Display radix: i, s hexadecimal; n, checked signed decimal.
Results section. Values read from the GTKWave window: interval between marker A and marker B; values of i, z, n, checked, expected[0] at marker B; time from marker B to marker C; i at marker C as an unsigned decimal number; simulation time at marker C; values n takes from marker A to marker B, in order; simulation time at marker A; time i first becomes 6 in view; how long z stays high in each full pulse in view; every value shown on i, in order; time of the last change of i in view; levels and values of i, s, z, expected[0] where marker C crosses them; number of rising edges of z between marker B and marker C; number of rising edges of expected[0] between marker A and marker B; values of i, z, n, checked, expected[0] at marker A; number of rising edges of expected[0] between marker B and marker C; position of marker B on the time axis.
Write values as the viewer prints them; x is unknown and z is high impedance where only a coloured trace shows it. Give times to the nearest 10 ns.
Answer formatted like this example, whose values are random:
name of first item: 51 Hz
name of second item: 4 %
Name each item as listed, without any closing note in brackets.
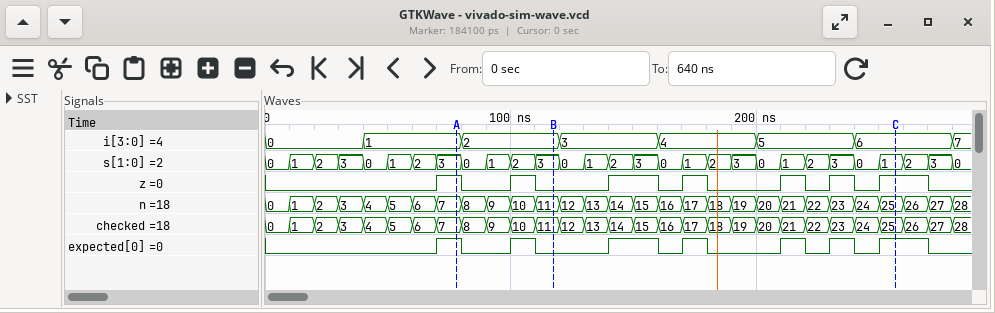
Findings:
interval between marker A and marker B: 40 ns
values of i, z, n, checked, expected[0] at marker B: i=2, z=0, n=11, checked=11, expected[0]=0
time from marker B to marker C: 140 ns
i at marker C as an unsigned decimal number: 6
simulation time at marker C: 260 ns
values n takes from marker A to marker B, in order: 7, 8, 9, 10, 11
simulation time at marker A: 80 ns
time i first becomes 6 in view: 240 ns
how long z stays high in each full pulse in view: 10 ns, 10 ns, 20 ns, 10 ns, 10 ns, 10 ns, 20 ns
every value shown on i, in order: 0, 1, 2, 3, 4, 5, 6, 7
time of the last change of i in view: 280 ns
levels and values of i, s, z, expected[0] where marker C crosses them: i=6, s=1, z=1, expected[0]=1
number of rising edges of z between marker B and marker C: 5
number of rising edges of expected[0] between marker A and marker B: 1
values of i, z, n, checked, expected[0] at marker A: i=1, z=1, n=7, checked=7, expected[0]=1
number of rising edges of expected[0] between marker B and marker C: 5
position of marker B on the time axis: 120 ns
